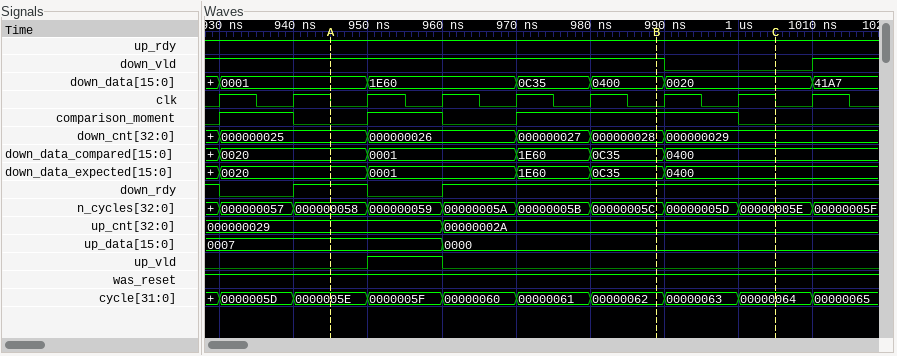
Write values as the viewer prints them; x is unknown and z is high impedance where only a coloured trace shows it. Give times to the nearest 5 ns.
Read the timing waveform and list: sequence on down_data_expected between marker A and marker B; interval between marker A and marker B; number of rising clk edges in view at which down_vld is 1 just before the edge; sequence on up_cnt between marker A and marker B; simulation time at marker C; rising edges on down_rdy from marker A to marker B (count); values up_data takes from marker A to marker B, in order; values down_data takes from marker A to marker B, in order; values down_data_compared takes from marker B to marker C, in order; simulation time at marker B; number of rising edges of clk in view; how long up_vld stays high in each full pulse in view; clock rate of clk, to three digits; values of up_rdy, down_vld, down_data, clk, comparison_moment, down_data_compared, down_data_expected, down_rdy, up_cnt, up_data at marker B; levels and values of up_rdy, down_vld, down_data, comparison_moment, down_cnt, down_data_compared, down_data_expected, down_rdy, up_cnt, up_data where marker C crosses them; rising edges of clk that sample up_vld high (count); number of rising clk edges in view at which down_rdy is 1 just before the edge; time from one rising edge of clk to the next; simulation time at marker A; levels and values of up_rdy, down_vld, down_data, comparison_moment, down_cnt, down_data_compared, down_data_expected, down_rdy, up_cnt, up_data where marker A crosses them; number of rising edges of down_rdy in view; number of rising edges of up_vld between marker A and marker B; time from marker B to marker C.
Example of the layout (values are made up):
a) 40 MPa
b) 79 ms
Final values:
a) 0020, 0001, 1E60, 0C35
b) 45 ns
c) 7
d) 000000029, 00000002A
e) 1005 ns
f) 1
g) 0007, 0000
h) 0001, 1E60, 0C35, 0400
i) 0C35, 0400
j) 990 ns
k) 9
l) 10 ns
m) 100 MHz
n) up_rdy=1, down_vld=1, down_data=0400, clk=0, comparison_moment=1, down_data_compared=0C35, down_data_expected=0C35, down_rdy=1, up_cnt=00000002A, up_data=0000
o) up_rdy=1, down_vld=0, down_data=0020, comparison_moment=0, down_cnt=000000029, down_data_compared=0400, down_data_expected=0400, down_rdy=1, up_cnt=00000002A, up_data=0000
p) 1
q) 7
r) 10 ns
s) 945 ns
t) up_rdy=1, down_vld=1, down_data=0001, comparison_moment=0, down_cnt=000000025, down_data_compared=0020, down_data_expected=0020, down_rdy=1, up_cnt=000000029, up_data=0007
u) 2
v) 1
w) 15 ns
